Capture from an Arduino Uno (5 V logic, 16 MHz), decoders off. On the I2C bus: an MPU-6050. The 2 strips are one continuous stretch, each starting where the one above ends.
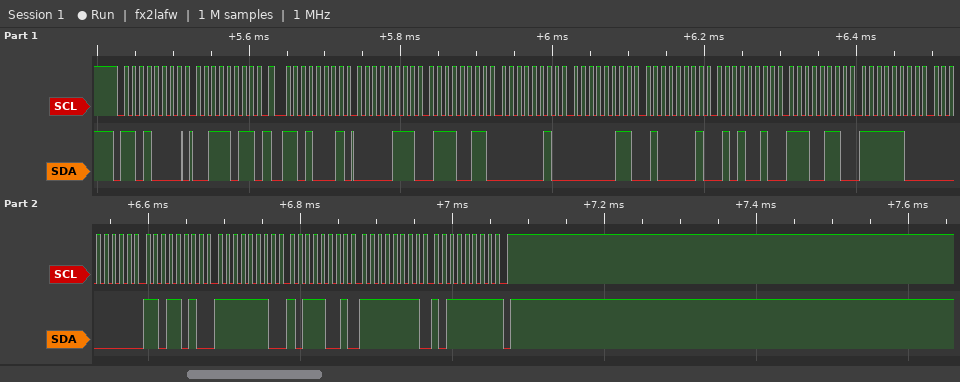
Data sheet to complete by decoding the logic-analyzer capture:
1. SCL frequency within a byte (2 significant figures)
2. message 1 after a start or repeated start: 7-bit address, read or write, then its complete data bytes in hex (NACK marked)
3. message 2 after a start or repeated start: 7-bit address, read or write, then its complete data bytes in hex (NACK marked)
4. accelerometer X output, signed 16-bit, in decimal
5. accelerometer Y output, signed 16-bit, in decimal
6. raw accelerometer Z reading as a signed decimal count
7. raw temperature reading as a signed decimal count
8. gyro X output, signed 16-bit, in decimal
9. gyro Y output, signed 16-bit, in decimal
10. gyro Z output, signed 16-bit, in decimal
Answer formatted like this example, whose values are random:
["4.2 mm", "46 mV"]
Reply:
["100 kHz", "0x68 write: 3B", "0x68 read: 07 73 02 03 41 52 E6 FC 00 DA FE B9 FF BF NACK", "1907", "515", "16722", "-6404", "218", "-327", "-65"]
